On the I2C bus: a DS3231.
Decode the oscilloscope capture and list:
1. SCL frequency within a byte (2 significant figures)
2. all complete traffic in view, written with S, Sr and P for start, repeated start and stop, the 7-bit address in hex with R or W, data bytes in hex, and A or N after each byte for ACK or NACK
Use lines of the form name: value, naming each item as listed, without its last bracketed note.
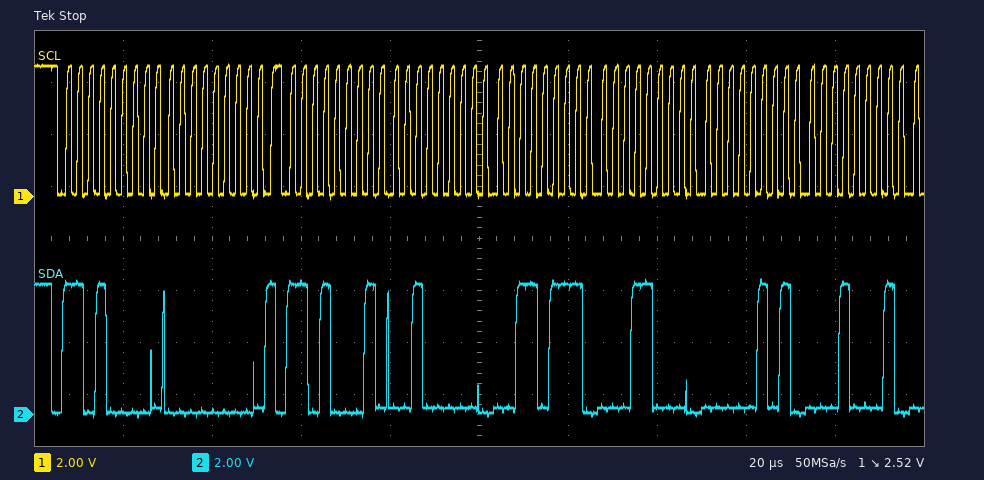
SCL frequency within a byte: 400 kHz
all complete traffic in view, written with S, Sr and P for start, repeated start and stop, the 7-bit address in hex with R or W, data bytes in hex, and A or N after each byte for ACK or NACK: S 68W A 00 A Sr 68R A 20 A 37 A 18 A 05 A 11 A
